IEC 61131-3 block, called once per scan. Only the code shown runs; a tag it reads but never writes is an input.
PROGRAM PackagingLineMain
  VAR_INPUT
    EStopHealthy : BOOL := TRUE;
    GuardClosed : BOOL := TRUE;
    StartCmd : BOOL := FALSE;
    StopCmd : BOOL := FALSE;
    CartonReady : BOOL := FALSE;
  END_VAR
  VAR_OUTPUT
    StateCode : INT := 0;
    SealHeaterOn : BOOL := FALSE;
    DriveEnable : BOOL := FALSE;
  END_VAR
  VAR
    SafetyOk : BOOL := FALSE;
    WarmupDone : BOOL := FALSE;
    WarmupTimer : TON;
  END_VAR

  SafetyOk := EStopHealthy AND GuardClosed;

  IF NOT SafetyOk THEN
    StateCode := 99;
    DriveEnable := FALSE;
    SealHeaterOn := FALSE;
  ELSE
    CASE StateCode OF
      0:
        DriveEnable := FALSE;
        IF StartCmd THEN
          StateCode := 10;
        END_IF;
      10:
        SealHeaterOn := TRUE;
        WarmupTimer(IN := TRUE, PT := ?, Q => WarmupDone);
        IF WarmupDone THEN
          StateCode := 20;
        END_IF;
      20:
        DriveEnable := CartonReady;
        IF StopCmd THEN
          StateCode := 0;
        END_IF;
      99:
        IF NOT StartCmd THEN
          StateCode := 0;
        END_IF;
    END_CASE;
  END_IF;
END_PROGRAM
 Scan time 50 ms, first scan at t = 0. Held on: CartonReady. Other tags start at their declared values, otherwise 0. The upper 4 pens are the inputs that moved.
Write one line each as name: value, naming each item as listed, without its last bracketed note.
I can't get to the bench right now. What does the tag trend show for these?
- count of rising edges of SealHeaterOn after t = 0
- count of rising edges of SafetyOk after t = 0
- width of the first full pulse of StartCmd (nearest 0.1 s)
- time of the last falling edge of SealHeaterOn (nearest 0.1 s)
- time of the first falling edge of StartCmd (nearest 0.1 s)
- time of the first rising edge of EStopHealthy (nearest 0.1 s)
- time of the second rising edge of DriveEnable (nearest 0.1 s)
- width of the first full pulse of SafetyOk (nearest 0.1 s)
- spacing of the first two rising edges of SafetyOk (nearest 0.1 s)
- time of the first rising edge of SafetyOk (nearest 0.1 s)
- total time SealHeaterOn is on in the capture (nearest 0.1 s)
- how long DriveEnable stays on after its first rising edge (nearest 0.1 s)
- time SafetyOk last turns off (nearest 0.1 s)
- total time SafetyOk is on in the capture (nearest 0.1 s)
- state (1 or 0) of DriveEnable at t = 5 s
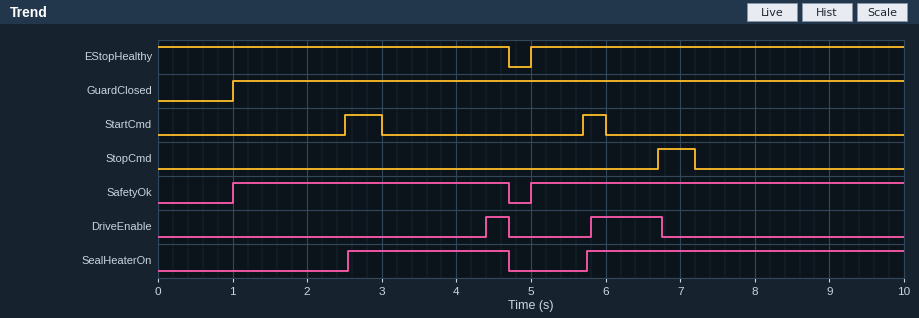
count of rising edges of SealHeaterOn after t = 0: 2
count of rising edges of SafetyOk after t = 0: 2
width of the first full pulse of StartCmd: 0.5 s
time of the last falling edge of SealHeaterOn: 4.7 s
time of the first falling edge of StartCmd: 3.0 s
time of the first rising edge of EStopHealthy: 5.0 s
time of the second rising edge of DriveEnable: 5.8 s
width of the first full pulse of SafetyOk: 3.7 s
spacing of the first two rising edges of SafetyOk: 4.0 s
time of the first rising edge of SafetyOk: 1.0 s
total time SealHeaterOn is on in the capture: 6.4 s
how long DriveEnable stays on after its first rising edge: 0.3 s
time SafetyOk last turns off: 4.7 s
total time SafetyOk is on in the capture: 8.7 s
state (1 or 0) of DriveEnable at t = 5 s: 0
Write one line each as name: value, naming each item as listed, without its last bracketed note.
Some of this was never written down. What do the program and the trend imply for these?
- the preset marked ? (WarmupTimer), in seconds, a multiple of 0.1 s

the preset marked ? (WarmupTimer), in seconds, a multiple of 0.1 s: 1.8 s
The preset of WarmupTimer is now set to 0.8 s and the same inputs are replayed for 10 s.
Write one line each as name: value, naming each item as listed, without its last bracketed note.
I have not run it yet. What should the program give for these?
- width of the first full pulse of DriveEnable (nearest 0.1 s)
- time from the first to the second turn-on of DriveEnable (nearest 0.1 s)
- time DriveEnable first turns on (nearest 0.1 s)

width of the first full pulse of DriveEnable: 1.3 s
time from the first to the second turn-on of DriveEnable: 2.4 s
time DriveEnable first turns on: 3.4 s
